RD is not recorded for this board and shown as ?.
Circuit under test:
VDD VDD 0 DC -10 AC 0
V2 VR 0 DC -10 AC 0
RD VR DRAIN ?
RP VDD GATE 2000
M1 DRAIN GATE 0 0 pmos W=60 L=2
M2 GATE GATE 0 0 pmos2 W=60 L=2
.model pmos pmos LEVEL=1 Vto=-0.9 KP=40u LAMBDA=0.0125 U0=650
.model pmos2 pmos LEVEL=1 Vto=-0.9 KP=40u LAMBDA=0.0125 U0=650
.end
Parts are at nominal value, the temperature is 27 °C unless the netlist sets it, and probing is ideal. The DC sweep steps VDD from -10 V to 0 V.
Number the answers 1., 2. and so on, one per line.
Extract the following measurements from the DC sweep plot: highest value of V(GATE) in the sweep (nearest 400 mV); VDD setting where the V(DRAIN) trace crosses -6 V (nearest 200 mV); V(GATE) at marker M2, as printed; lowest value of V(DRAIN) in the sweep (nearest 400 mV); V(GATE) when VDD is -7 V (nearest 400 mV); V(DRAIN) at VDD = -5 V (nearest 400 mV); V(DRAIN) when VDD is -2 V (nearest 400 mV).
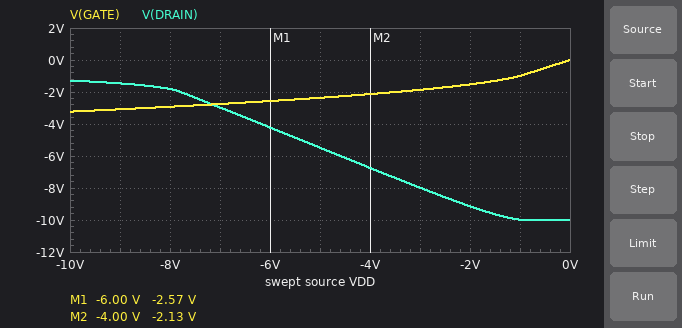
1. 0 V
2. -4.6 V
3. -2.13 V
4. -10.0 V
5. -2.8 V
6. -5.6 V
7. -9.2 V
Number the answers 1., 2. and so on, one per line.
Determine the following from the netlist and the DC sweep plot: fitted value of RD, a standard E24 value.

1. 3.3 kΩ
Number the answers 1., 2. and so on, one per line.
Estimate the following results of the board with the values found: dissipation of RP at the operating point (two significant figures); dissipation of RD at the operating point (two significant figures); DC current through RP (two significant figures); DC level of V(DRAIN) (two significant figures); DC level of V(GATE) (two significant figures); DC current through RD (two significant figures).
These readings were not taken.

1. 23 mW
2. 23 mW
3. 3.4 mA
4. -1.3 V
5. -3.2 V
6. 2.6 mA
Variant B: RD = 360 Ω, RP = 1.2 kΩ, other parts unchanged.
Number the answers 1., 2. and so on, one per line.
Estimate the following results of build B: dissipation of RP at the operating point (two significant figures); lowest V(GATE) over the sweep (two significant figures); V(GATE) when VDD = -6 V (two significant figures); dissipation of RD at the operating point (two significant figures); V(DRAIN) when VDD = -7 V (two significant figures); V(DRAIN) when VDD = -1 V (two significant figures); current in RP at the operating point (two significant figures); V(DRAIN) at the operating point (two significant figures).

1. 32 mW
2. -3.8 V
3. -2.9 V
4. 11 mW
5. -8.8 V
6. -10 V
7. 5.2 mA
8. -8.0 V
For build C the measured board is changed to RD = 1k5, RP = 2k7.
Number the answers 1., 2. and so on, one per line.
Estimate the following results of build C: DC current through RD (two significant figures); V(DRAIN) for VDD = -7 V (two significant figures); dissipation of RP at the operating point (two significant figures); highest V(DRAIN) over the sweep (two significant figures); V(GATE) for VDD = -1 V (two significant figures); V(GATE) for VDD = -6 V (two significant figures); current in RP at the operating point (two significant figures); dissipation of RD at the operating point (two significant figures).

1. 2.7 mA
2. -7.4 V
3. 18 mW
4. -5.9 V
5. -990 mV
6. -2.4 V
7. 2.6 mA
8. 11 mW
